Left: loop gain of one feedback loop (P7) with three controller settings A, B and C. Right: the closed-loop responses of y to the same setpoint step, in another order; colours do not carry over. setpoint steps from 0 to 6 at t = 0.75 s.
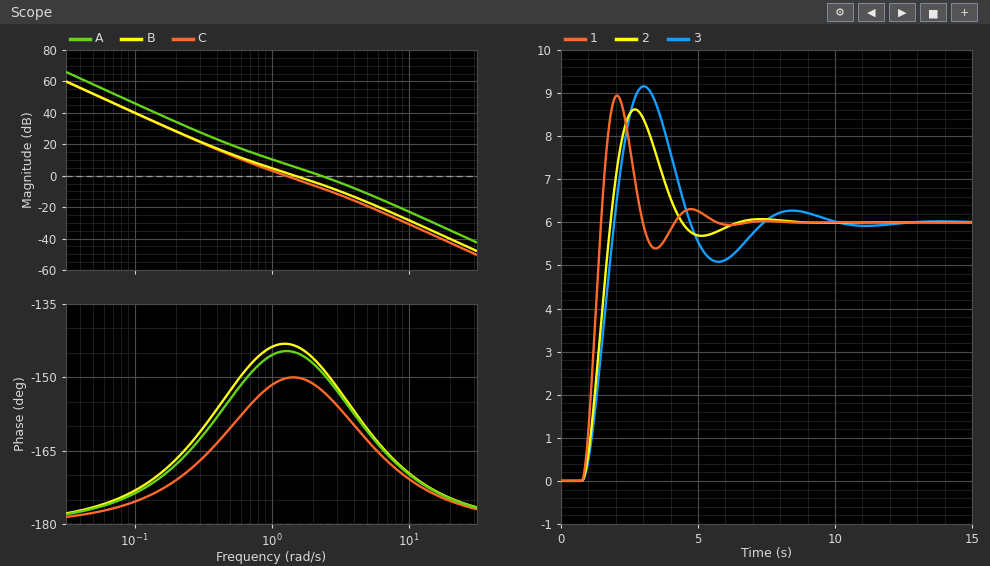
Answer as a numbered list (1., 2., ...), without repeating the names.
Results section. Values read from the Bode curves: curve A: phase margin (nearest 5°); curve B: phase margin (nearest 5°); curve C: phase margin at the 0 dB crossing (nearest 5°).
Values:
1. 30°
2. 35°
3. 30°
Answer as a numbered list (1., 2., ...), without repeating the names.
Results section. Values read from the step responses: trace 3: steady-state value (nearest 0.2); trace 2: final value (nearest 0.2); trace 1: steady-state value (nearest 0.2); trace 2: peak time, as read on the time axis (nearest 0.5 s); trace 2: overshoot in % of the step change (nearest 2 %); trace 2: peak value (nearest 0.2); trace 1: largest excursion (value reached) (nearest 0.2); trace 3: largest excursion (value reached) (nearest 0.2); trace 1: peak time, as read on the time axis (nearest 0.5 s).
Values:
1. 6.0
2. 6.0
3. 6.0
4. 2.5 s
5. 44 %
6. 8.6
7. 9.0
8. 9.2
9. 2.0 s
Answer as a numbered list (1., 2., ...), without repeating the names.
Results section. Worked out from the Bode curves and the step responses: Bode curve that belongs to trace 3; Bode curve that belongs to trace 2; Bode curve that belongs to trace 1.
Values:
1. C
2. B
3. A
